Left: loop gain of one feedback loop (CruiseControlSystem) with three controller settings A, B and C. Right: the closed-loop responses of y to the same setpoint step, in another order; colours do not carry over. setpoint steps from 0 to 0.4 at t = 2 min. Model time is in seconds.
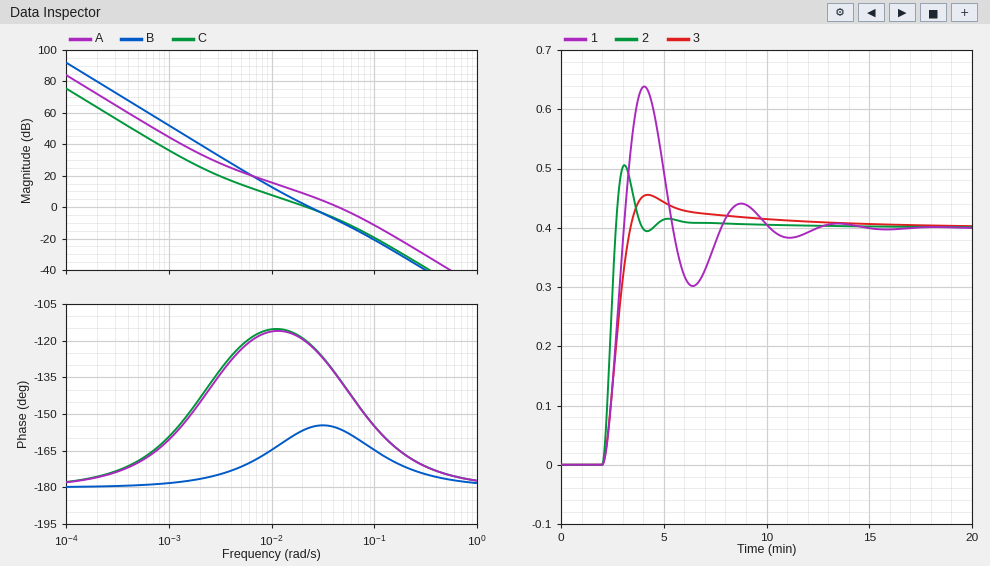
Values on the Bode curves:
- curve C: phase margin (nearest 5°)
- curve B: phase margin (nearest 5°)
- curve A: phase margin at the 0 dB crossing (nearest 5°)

60°
25°
45°
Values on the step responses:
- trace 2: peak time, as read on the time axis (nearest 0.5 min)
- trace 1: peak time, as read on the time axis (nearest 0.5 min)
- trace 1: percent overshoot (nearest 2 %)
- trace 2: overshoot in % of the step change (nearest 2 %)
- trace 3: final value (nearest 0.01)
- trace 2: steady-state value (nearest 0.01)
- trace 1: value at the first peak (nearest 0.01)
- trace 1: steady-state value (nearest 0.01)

3.0 min
4.0 min
60 %
26 %
0.40
0.40
0.64
0.40
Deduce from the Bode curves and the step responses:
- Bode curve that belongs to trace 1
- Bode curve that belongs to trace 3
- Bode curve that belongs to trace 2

B
C
A
